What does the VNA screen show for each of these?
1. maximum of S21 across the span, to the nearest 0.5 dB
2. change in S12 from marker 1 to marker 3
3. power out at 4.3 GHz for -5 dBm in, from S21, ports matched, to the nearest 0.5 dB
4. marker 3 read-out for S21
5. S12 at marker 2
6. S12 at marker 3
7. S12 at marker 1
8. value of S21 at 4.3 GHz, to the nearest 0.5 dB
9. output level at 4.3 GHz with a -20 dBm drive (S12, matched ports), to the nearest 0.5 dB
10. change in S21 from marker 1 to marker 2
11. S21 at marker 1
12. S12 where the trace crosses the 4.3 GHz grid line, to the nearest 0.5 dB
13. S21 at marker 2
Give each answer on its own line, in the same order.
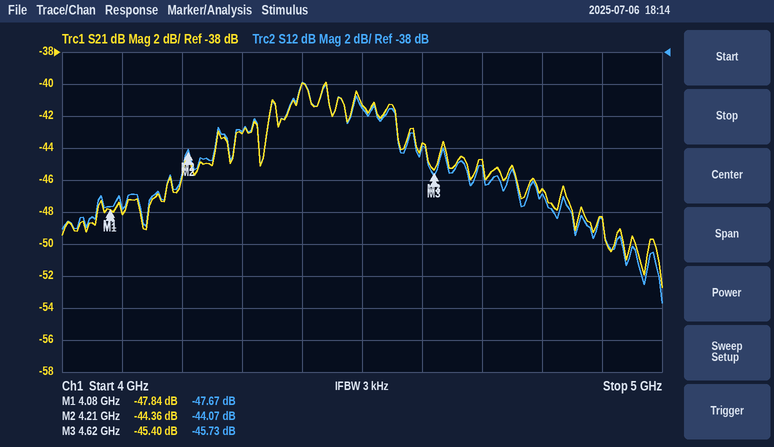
-40.0 dB
1.94 dB
-48.0 dBm
-45.40 dB
-44.07 dB
-45.73 dB
-47.67 dB
-43.0 dB
-63.0 dBm
3.48 dB
-47.84 dB
-43.0 dB
-44.36 dB
